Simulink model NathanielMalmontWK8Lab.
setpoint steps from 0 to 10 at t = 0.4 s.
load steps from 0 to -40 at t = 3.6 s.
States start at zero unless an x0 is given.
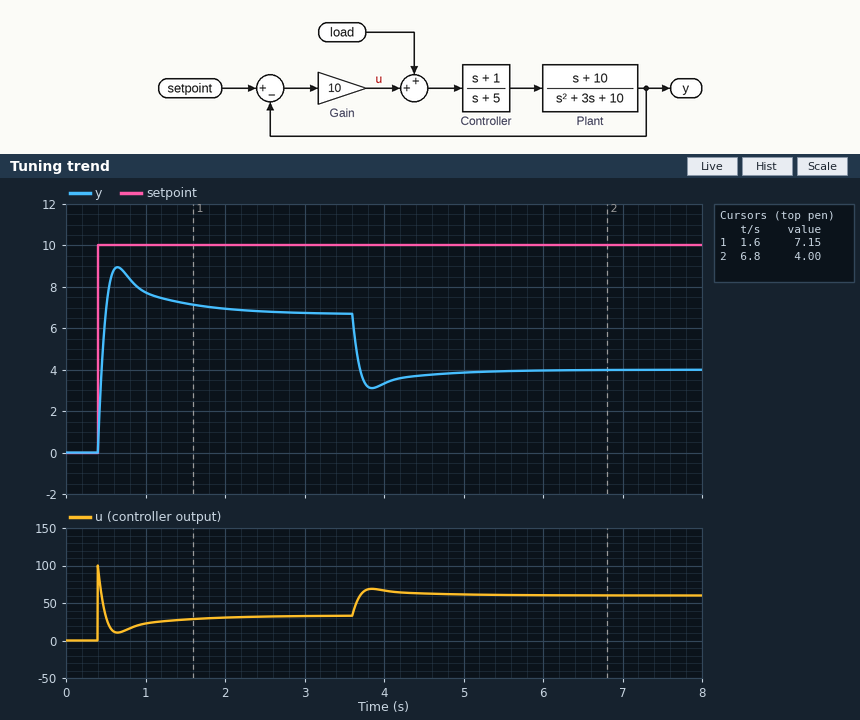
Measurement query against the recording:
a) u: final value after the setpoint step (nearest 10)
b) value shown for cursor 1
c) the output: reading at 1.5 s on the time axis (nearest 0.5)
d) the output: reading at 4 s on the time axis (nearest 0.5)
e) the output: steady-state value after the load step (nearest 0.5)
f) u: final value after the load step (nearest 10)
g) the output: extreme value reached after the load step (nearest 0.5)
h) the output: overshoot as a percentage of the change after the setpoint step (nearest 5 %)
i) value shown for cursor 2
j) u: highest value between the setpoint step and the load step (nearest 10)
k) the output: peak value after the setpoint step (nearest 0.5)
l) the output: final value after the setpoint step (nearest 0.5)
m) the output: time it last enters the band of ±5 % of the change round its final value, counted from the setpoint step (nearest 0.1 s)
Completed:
30
7.15
7.0
3.5
4.0
60
3.0
35 %
4.00
100
9.0
6.5
1.5 s
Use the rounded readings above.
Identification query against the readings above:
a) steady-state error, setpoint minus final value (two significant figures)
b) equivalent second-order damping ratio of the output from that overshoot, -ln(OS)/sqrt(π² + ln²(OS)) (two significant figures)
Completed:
3.5
0.32
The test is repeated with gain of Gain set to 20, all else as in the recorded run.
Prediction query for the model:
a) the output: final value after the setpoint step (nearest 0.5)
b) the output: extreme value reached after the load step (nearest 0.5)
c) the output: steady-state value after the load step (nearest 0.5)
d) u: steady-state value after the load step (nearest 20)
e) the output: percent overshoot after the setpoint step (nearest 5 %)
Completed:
8.0
6.0
6.5
80
20 %
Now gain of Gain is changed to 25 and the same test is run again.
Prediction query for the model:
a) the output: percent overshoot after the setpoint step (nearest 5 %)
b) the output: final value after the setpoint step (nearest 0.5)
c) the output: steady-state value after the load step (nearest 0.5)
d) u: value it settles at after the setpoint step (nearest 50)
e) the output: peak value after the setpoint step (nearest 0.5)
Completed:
20 %
8.5
7.0
50
10.0
